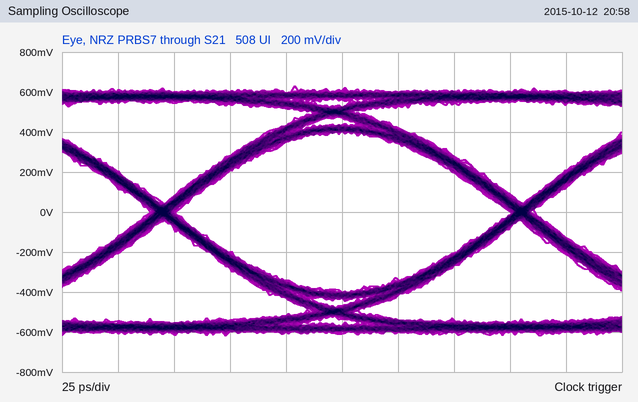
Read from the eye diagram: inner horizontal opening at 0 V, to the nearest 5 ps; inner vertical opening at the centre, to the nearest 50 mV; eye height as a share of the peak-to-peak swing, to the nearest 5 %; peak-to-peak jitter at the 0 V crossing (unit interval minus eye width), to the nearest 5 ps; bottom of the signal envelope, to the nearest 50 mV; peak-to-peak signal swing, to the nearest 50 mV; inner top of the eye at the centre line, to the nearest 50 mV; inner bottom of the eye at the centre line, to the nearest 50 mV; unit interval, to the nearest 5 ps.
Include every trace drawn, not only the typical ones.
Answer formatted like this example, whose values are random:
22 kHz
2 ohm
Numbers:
150 ps
800 mV
65 %
10 ps
-600 mV
1.25 V
400 mV
-400 mV
160 ps
